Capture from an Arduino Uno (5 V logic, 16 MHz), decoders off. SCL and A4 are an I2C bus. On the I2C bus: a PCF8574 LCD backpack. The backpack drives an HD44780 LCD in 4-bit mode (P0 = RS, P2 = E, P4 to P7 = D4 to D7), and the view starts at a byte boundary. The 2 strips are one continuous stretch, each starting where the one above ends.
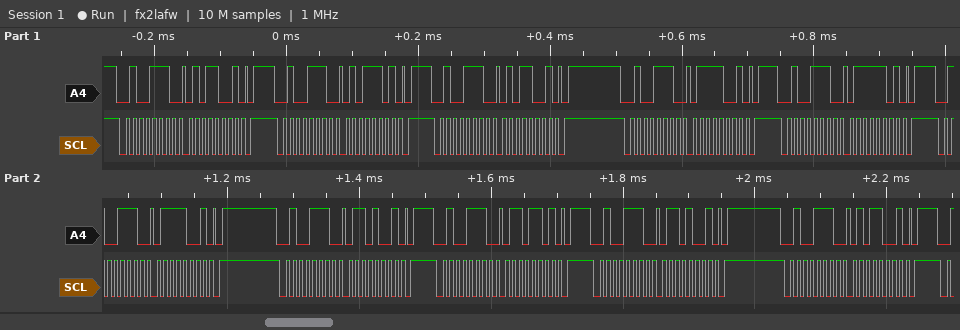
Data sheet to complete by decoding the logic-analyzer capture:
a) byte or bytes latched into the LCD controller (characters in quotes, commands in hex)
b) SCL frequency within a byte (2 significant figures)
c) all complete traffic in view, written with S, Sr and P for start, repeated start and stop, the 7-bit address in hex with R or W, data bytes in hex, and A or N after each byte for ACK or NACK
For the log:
'W'
100 kHz
S 27W A 59 A P S 27W A 5D A P S 27W A 59 A P S 27W A 79 A P S 27W A 7D A P S 27W A 79 A P S 27W A 69 A P S 27W A 6D A P S 27W A 69 A P S 27W A 59 A P
